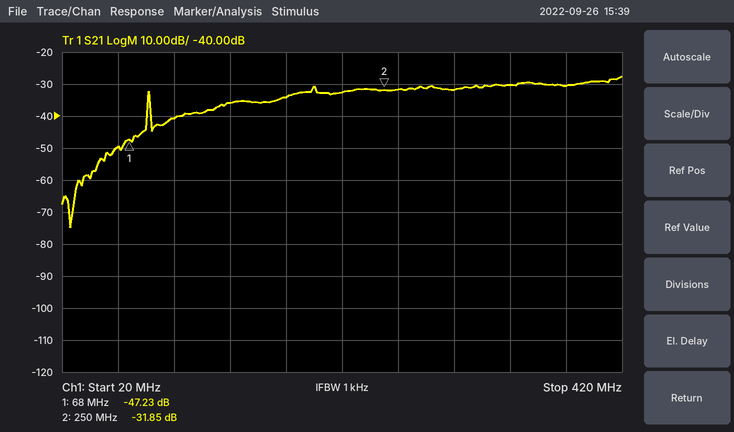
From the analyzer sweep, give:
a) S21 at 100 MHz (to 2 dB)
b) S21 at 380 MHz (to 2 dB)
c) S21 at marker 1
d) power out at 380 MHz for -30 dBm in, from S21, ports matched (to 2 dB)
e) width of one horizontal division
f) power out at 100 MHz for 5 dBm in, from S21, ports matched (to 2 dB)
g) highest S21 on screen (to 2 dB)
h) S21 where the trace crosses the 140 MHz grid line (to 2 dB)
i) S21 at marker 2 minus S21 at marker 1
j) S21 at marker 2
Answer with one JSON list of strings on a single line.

["-40 dB", "-30 dB", "-47.23 dB", "-60 dBm", "40 MHz", "-36 dBm", "-28 dB", "-36 dB", "15.38 dB", "-31.85 dB"]
